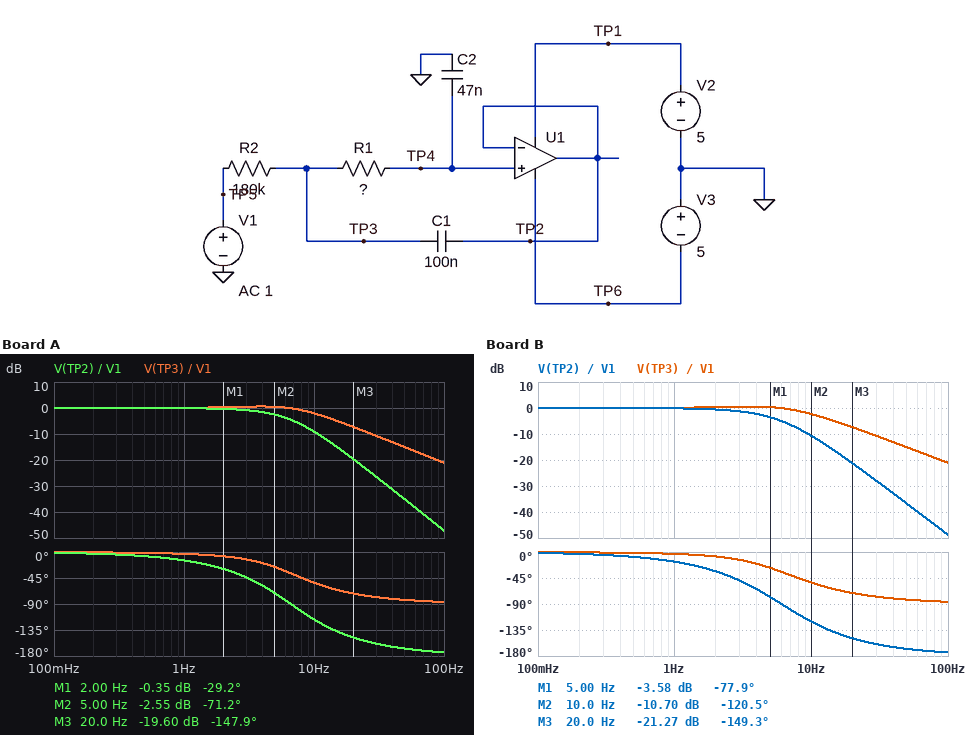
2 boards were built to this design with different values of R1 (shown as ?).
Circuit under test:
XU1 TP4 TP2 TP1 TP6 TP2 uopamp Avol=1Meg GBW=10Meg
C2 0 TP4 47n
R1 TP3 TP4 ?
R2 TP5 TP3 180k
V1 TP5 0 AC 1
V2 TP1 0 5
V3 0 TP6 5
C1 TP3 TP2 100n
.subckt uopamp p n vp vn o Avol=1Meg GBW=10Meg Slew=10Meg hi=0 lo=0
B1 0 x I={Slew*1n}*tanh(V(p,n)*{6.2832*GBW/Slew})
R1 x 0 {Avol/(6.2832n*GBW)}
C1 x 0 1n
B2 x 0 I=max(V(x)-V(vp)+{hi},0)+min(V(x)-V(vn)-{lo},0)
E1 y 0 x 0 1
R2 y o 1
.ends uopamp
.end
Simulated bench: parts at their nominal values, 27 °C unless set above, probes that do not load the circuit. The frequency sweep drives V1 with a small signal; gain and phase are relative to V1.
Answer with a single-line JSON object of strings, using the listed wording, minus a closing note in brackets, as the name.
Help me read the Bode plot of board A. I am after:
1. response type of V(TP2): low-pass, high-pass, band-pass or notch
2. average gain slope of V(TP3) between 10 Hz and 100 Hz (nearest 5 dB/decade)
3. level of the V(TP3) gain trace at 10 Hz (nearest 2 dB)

{"response type of V(TP2): low-pass, high-pass, band-pass or notch": "low-pass", "average gain slope of V(TP3) between 10 Hz and 100 Hz": "-20 dB/decade", "level of the V(TP3) gain trace at 10 Hz": "-2 dB"}
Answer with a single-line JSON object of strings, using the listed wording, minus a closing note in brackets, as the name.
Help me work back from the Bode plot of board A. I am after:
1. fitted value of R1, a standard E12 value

{"fitted value of R1, a standard E12 value": "680 kΩ"}
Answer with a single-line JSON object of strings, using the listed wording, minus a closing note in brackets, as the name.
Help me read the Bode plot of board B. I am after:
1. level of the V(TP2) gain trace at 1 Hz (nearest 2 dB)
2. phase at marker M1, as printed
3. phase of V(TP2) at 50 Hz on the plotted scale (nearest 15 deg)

{"level of the V(TP2) gain trace at 1 Hz": "0 dB", "phase at marker M1, as printed": "-77.9 deg", "phase of V(TP2) at 50 Hz on the plotted scale": "-165 deg"}
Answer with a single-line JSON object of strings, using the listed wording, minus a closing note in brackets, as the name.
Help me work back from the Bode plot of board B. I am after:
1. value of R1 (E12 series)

{"value of R1": "820 kΩ"}
